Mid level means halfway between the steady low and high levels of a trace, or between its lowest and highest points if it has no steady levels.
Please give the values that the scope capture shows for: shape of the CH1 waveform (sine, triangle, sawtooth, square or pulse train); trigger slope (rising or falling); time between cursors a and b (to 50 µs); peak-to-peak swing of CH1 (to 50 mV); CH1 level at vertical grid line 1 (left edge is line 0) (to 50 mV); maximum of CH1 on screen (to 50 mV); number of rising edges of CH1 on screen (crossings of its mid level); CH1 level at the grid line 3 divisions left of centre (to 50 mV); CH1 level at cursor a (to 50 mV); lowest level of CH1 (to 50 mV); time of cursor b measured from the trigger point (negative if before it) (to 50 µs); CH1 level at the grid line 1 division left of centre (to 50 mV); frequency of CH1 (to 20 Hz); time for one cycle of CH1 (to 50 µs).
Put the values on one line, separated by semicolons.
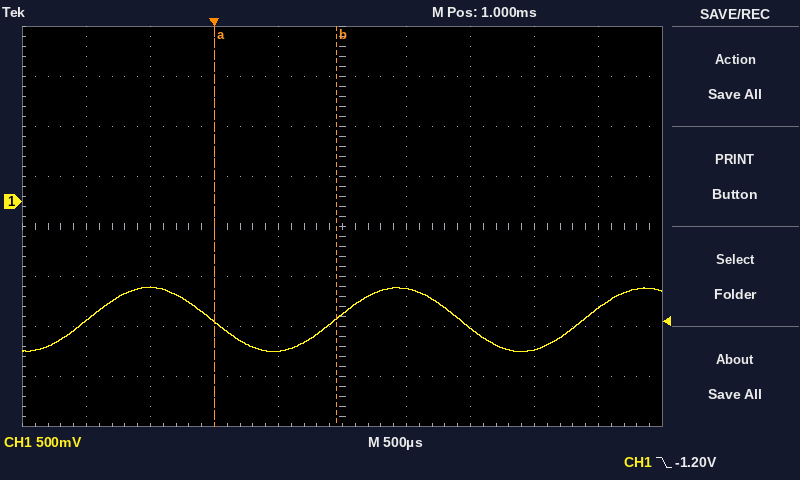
sine; falling; 950 µs; 650 mV; -1.20 V; -850 mV; 3; -850 mV; -1.20 V; -1.50 V; +950 µs; -1.50 V; 520 Hz; 1.95 ms
